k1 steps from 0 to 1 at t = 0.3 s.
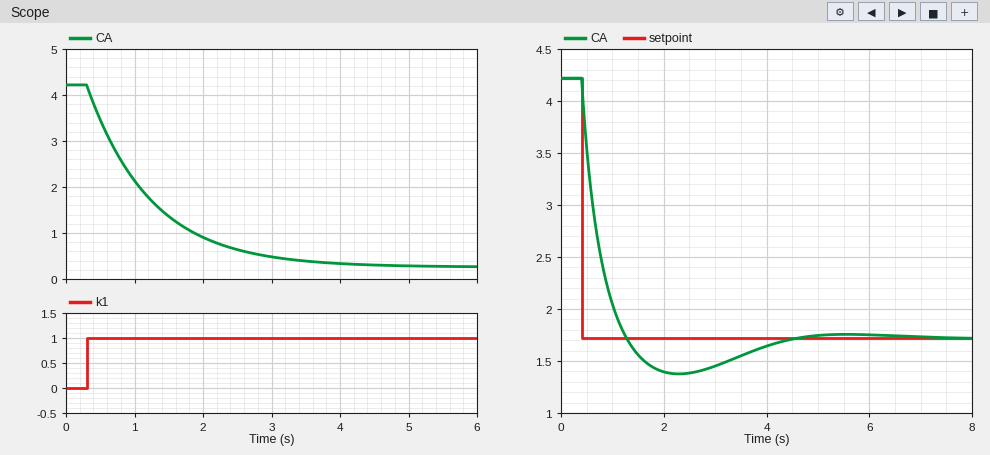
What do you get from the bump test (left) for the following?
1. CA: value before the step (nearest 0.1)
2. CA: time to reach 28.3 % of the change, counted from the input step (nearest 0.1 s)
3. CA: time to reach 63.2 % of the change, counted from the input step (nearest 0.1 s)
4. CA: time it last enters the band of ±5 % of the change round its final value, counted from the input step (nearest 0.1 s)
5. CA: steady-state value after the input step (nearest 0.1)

4.2
0.3 s
0.9 s
2.8 s
0.3
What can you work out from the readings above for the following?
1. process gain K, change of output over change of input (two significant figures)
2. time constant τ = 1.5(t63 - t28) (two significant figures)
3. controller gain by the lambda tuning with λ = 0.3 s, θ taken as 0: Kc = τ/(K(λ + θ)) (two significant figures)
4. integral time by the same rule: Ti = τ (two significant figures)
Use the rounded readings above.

-3.9
0.90 s
-0.77
0.90 s
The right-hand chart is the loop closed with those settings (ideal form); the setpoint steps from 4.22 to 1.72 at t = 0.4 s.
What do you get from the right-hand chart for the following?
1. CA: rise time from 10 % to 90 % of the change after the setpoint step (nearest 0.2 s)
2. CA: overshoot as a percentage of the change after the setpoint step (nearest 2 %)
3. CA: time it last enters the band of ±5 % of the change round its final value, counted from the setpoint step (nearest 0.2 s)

0.6 s
14 %
3.4 s
